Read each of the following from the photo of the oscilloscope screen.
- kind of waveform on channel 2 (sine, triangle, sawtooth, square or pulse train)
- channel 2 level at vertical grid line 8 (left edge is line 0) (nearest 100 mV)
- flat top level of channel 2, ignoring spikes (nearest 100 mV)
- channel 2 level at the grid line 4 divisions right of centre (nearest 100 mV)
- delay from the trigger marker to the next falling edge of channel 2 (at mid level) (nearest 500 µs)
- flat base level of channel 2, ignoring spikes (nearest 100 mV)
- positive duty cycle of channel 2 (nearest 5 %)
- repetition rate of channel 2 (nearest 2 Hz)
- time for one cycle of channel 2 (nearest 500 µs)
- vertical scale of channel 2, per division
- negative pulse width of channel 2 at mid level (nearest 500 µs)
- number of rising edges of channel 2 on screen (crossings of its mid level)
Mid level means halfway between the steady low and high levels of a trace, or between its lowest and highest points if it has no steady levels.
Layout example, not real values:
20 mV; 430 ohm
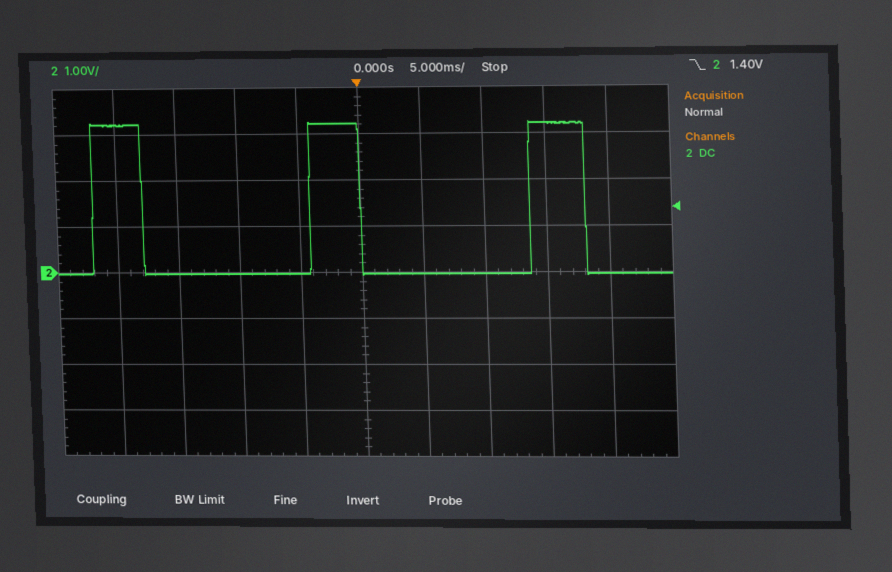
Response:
pulse train; 3.2 V; 3.2 V; 0.0 V; 18.0 ms; 0.0 V; 25 %; 56 Hz; 18.0 ms; 1 V; 13.5 ms; 3
